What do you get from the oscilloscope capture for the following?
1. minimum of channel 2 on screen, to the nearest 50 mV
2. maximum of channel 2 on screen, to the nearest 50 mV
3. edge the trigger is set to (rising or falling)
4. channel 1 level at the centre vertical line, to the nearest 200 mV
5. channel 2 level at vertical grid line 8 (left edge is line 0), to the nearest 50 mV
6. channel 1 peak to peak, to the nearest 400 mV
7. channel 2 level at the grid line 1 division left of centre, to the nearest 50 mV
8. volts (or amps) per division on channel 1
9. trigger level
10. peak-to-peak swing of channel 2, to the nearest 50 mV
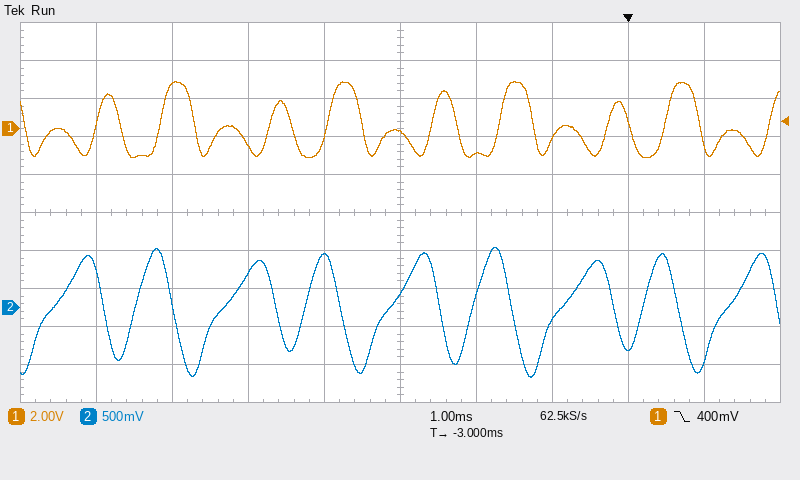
-900 mV
800 mV
falling
-200 mV
-550 mV
4.0 V
700 mV
2 V
400 mV
1.70 V
